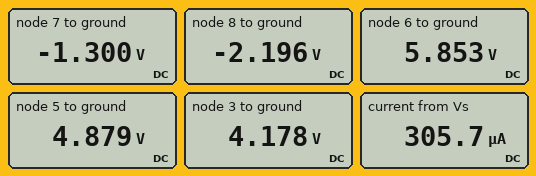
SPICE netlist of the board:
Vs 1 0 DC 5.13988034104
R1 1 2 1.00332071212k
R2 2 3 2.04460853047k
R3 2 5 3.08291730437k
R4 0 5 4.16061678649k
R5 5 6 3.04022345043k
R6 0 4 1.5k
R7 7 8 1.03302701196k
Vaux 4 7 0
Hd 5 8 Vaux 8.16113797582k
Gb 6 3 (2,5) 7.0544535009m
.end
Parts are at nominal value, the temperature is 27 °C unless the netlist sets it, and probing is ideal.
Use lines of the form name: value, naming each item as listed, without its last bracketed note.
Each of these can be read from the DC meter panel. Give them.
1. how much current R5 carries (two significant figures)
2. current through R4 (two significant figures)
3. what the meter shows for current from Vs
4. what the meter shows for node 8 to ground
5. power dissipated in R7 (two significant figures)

how much current R5 carries: 320 µA
current through R4: 1.2 mA
what the meter shows for current from Vs: 305.7 µA
what the meter shows for node 8 to ground: -2.196 V
power dissipated in R7: 780 µW
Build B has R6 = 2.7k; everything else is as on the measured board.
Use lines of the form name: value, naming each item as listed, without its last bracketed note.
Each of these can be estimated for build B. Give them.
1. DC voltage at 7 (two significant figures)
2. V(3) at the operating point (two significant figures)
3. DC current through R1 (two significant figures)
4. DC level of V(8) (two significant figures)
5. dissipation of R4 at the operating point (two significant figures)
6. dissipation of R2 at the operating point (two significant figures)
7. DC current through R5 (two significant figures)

DC voltage at 7: -3.1 V
V(3) at the operating point: 4.9 V
DC current through R1: 74 µA
DC level of V(8): -4.3 V
dissipation of R4 at the operating point: 6.2 mW
dissipation of R2 at the operating point: 12 µW
DC current through R5: 77 µA
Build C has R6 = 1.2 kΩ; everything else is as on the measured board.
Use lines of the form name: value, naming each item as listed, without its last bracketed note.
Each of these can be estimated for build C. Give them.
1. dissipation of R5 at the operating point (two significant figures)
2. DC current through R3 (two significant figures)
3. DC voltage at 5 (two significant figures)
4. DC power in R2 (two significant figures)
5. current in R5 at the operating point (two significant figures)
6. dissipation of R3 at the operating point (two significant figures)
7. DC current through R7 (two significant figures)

dissipation of R5 at the operating point: 400 µW
DC current through R3: 17 µA
DC voltage at 5: 4.8 V
DC power in R2: 270 µW
current in R5 at the operating point: 360 µA
dissipation of R3 at the operating point: 860 nW
DC current through R7: 820 µA
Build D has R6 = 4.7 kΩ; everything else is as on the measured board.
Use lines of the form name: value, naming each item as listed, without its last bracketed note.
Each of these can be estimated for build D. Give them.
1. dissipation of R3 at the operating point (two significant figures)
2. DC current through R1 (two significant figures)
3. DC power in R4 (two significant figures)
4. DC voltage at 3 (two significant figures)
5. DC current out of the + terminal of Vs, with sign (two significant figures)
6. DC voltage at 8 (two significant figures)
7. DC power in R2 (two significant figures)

dissipation of R3 at the operating point: 7.6 µW
DC current through R1: 1.0 mA
DC power in R4: 8.7 mW
DC voltage at 3: 8.4 V
DC current out of the + terminal of Vs, with sign: -1.0 mA
DC voltage at 8: -14 V
DC power in R2: 2.4 mW
